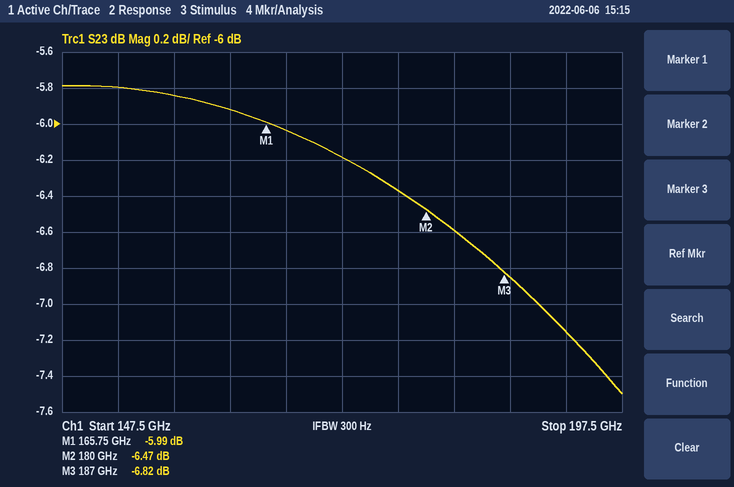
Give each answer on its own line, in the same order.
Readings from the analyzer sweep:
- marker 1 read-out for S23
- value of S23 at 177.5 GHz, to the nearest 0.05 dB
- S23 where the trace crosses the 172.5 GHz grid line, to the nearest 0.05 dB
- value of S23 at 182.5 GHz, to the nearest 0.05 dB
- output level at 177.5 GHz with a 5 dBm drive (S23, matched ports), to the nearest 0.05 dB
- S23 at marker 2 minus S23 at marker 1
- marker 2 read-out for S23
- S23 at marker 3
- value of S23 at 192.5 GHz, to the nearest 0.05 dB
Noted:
-5.99 dB
-6.35 dB
-6.20 dB
-6.60 dB
-1.35 dBm
-0.48 dB
-6.47 dB
-6.82 dB
-7.15 dB
